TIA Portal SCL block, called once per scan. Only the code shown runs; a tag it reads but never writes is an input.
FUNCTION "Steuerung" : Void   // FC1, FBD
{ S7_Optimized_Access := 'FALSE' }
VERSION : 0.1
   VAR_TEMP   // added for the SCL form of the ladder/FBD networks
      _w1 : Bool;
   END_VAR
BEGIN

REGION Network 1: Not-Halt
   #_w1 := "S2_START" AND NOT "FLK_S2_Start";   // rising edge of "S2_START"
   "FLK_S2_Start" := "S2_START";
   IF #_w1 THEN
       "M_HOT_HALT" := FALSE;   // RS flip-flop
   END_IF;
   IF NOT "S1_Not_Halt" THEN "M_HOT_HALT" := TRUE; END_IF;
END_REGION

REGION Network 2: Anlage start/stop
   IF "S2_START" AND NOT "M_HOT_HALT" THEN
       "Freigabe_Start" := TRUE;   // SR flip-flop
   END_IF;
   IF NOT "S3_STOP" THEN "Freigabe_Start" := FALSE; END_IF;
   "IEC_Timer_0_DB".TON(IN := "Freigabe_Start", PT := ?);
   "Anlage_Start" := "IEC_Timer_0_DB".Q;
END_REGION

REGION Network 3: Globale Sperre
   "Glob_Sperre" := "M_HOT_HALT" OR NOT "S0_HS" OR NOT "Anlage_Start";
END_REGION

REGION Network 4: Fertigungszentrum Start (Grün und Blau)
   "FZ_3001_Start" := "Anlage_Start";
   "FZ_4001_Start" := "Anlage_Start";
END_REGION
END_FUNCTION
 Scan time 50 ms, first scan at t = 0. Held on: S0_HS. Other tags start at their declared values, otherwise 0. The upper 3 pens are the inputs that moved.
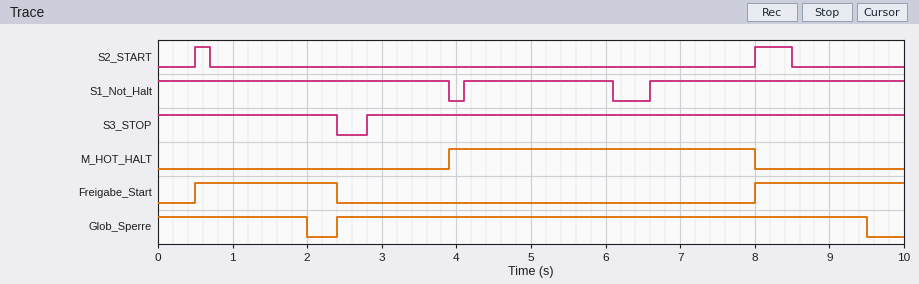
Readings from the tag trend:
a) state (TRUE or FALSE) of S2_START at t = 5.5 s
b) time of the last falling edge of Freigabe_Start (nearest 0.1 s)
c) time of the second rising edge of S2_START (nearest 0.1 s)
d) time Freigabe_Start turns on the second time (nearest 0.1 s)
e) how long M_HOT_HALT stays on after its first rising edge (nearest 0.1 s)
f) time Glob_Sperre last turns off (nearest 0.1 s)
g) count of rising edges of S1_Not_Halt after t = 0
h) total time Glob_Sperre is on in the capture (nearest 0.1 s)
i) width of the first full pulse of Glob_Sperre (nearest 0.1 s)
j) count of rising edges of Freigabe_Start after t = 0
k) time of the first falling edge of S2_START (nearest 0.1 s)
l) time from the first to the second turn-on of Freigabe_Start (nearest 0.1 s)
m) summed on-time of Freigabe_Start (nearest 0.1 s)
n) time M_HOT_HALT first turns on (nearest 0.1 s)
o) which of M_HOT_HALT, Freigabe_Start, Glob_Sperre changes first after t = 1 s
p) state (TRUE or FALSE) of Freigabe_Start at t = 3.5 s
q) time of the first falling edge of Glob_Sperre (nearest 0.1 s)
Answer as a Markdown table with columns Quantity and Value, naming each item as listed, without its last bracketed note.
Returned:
| Quantity | Value |
|---|---|
| state (TRUE or FALSE) of S2_START at t = 5.5 s | FALSE |
| time of the last falling edge of Freigabe_Start | 2.4 s |
| time of the second rising edge of S2_START | 8.0 s |
| time Freigabe_Start turns on the second time | 8.0 s |
| how long M_HOT_HALT stays on after its first rising edge | 4.1 s |
| time Glob_Sperre last turns off | 9.5 s |
| count of rising edges of S1_Not_Halt after t = 0 | 2 |
| total time Glob_Sperre is on in the capture | 9.1 s |
| width of the first full pulse of Glob_Sperre | 7.1 s |
| count of rising edges of Freigabe_Start after t = 0 | 2 |
| time of the first falling edge of S2_START | 0.7 s |
| time from the first to the second turn-on of Freigabe_Start | 7.5 s |
| summed on-time of Freigabe_Start | 3.9 s |
| time M_HOT_HALT first turns on | 3.9 s |
| which of M_HOT_HALT, Freigabe_Start, Glob_Sperre changes first after t = 1 s | Glob_Sperre |
| state (TRUE or FALSE) of Freigabe_Start at t = 3.5 s | FALSE |
| time of the first falling edge of Glob_Sperre | 2.0 s |
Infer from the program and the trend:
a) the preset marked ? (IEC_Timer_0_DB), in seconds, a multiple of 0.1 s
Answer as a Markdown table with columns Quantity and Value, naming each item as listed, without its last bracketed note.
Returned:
| Quantity | Value |
|---|---|
| the preset marked ? (IEC_Timer_0_DB), in seconds, a multiple of 0.1 s | 1.5 s |
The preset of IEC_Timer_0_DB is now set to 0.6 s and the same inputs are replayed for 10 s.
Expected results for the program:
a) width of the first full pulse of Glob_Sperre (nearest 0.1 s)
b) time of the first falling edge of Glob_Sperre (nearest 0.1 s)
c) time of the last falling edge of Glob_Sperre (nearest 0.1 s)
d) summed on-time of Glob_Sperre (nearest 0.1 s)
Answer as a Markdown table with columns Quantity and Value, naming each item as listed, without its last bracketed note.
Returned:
| Quantity | Value |
|---|---|
| width of the first full pulse of Glob_Sperre | 6.2 s |
| time of the first falling edge of Glob_Sperre | 1.1 s |
| time of the last falling edge of Glob_Sperre | 8.6 s |
| summed on-time of Glob_Sperre | 7.3 s |
